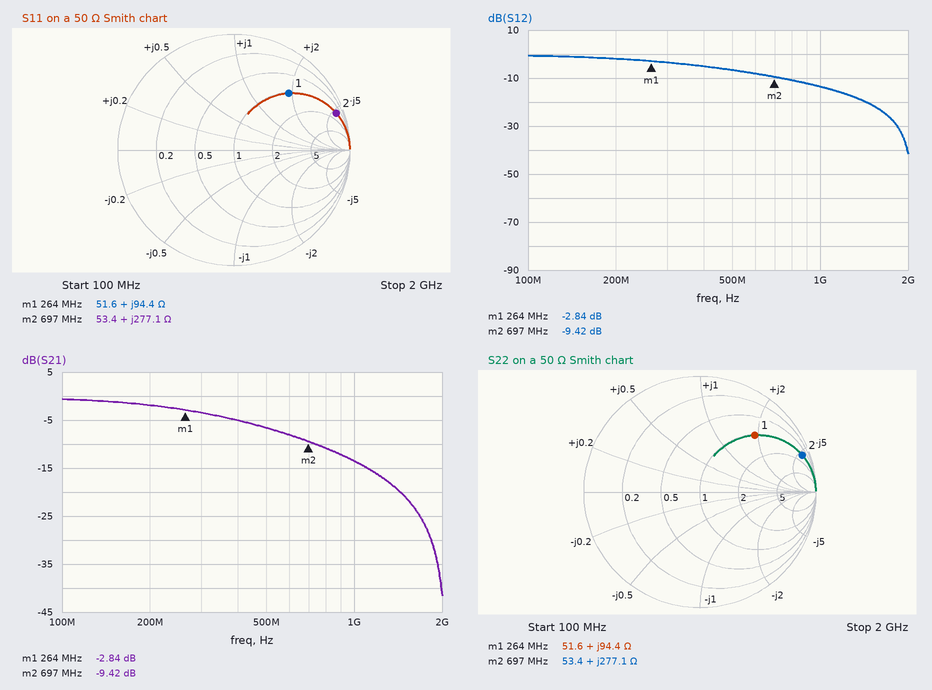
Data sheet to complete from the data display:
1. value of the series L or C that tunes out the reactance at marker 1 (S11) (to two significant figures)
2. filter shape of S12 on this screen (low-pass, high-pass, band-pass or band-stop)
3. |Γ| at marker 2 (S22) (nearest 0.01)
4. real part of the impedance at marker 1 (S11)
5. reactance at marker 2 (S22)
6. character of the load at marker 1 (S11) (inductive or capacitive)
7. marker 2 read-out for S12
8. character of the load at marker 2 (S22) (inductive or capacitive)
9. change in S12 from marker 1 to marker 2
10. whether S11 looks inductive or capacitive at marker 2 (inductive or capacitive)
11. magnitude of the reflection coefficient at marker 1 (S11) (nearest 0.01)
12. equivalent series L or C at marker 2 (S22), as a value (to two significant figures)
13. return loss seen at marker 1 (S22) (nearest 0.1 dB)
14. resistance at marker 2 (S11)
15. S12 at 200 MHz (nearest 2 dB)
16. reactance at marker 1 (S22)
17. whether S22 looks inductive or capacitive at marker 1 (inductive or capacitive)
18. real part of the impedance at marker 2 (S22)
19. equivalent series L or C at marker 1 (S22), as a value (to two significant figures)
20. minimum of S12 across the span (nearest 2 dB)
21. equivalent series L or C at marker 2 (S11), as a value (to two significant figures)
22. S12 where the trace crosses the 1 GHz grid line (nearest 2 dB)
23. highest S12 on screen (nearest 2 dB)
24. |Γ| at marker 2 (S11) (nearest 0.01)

6.4 pF
low-pass
0.94
51.6 Ω
+277.1 Ω
inductive
-9.42 dB
inductive
-6.58 dB
inductive
0.68
63 nH
3.3 dB
53.4 Ω
-2 dB
+94.4 Ω
inductive
53.4 Ω
57 nH
-42 dB
63 nH
-14 dB
0 dB
0.94
